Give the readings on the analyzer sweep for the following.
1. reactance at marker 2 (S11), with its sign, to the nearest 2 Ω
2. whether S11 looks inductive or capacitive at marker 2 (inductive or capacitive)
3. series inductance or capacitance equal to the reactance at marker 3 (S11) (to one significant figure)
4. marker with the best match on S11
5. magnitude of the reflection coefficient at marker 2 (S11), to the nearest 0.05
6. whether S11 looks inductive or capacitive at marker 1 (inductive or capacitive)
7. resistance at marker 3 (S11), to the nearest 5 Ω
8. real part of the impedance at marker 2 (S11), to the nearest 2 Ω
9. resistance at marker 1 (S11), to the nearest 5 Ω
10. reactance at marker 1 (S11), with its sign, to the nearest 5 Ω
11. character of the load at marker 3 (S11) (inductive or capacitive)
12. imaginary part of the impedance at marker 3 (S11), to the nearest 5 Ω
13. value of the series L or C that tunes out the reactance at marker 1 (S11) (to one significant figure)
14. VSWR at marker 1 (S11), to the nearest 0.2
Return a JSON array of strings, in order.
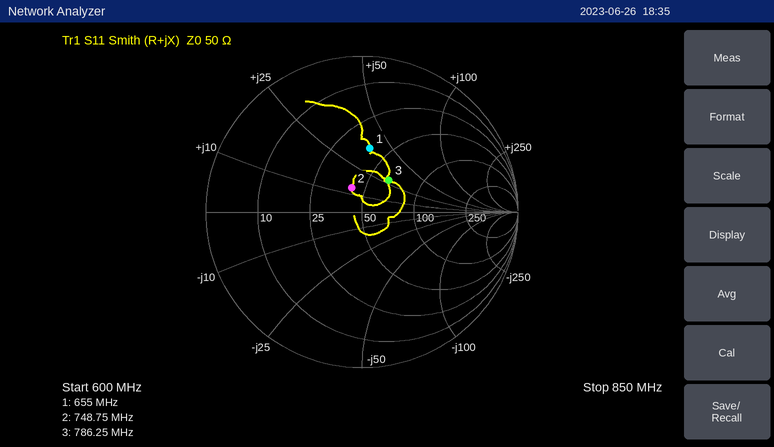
["+14 Ω", "inductive", "6 nH", "marker 2", "0.15", "inductive", "65 Ω", "42 Ω", "40 Ω", "+40 Ω", "inductive", "+30 Ω", "6 pF", "2.4"]
